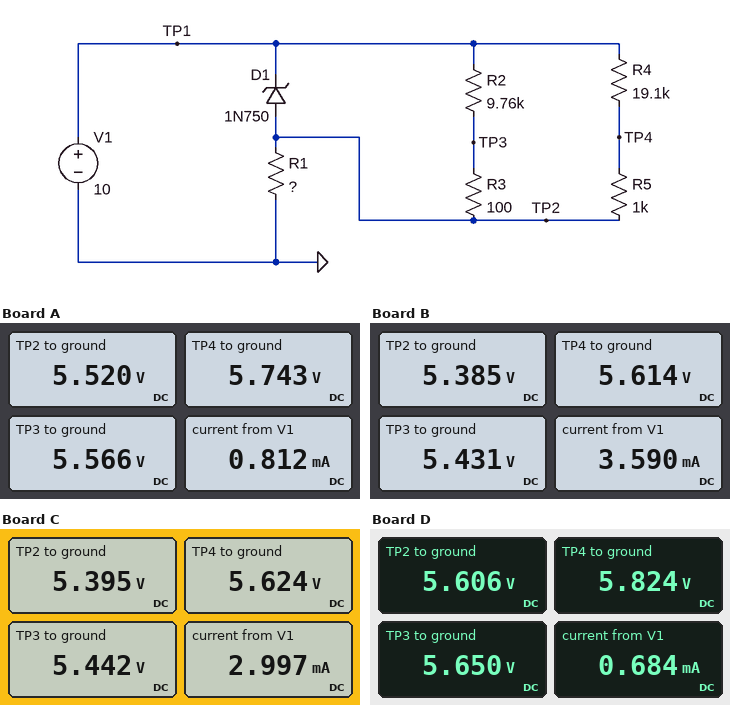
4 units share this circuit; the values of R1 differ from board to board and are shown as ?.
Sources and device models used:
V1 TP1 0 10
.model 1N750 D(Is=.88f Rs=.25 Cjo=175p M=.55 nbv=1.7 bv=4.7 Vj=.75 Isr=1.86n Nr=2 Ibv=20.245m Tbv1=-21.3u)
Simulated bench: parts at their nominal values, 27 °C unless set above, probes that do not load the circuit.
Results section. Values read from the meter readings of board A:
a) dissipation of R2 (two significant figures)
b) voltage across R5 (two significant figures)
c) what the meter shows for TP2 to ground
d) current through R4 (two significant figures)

2.0 mW
220 mV
5.520 V
220 µA
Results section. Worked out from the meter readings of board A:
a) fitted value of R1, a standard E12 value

6.8 kΩ
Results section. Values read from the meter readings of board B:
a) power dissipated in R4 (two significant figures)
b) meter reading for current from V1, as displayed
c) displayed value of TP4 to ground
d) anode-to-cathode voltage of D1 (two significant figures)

1.0 mW
3.590 mA
5.614 V
-4.6 V
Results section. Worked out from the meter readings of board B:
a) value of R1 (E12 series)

1.5 kΩ
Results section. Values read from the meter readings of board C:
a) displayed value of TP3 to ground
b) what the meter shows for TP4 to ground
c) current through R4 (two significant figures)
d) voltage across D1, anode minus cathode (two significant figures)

5.442 V
5.624 V
230 µA
-4.6 V
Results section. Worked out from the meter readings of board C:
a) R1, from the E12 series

1.8 kΩ
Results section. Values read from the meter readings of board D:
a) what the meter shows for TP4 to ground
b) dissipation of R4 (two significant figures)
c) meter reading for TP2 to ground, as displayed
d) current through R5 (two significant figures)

5.824 V
910 µW
5.606 V
220 µA
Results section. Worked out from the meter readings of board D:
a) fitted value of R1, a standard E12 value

8.2 kΩ
